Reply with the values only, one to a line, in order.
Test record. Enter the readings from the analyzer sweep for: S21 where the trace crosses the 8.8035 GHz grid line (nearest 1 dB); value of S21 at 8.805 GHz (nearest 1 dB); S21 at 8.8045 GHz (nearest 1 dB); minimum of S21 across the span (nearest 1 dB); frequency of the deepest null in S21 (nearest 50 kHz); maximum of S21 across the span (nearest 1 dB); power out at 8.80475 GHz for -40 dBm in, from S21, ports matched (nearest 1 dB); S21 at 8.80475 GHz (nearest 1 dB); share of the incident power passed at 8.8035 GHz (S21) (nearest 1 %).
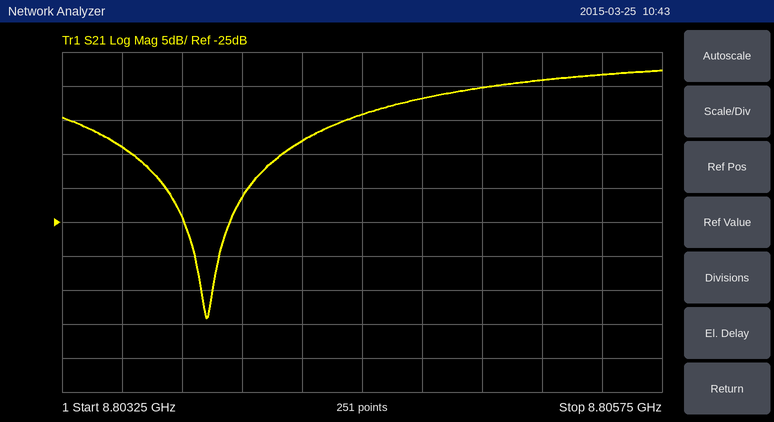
-14 dB
-5 dB
-9 dB
-39 dB
8.80385 GHz
-3 dB
-47 dBm
-7 dB
4 %
